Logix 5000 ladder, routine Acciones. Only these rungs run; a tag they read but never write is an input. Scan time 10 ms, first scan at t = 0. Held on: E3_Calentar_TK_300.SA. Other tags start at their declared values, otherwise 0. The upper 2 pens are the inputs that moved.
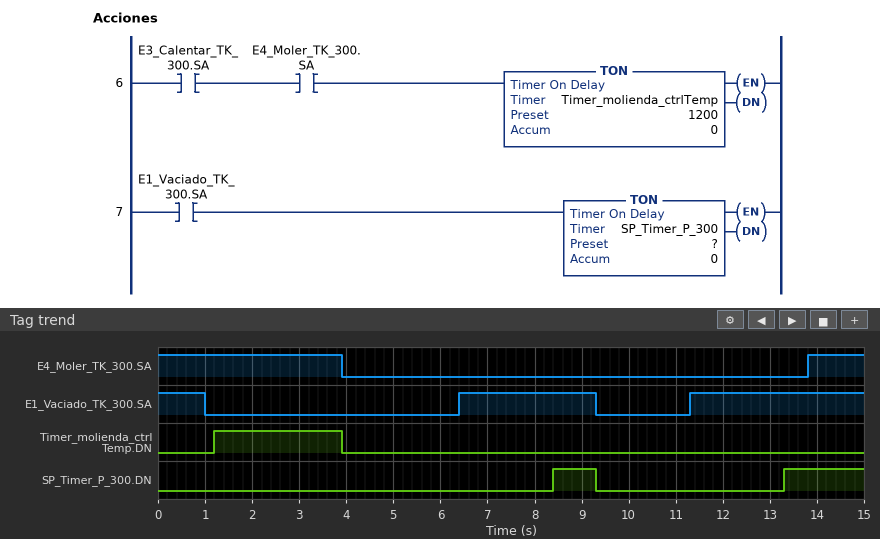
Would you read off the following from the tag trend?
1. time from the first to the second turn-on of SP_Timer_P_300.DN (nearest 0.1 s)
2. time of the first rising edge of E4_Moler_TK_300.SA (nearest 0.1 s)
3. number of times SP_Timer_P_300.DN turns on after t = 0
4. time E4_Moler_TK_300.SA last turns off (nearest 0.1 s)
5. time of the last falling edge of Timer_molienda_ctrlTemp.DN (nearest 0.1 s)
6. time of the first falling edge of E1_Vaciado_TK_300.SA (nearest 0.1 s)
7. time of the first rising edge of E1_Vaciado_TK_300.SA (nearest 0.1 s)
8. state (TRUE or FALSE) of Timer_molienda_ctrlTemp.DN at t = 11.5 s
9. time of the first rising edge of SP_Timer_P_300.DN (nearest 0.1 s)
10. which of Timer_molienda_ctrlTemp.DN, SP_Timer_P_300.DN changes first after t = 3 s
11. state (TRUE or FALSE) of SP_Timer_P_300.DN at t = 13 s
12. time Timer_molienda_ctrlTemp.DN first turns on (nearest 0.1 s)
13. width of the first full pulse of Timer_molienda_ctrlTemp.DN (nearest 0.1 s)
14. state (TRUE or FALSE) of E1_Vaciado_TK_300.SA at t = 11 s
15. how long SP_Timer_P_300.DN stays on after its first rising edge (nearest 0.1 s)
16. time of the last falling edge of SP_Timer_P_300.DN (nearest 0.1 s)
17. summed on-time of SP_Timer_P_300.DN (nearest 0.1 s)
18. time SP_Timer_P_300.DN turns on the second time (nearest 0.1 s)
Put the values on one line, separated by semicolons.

4.9 s; 13.8 s; 2; 3.9 s; 3.9 s; 1.0 s; 6.4 s; FALSE; 8.4 s; Timer_molienda_ctrlTemp.DN; FALSE; 1.2 s; 2.7 s; FALSE; 0.9 s; 9.3 s; 2.6 s; 13.3 s
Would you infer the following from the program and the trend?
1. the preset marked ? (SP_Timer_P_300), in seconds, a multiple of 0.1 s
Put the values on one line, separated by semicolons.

2.0 s
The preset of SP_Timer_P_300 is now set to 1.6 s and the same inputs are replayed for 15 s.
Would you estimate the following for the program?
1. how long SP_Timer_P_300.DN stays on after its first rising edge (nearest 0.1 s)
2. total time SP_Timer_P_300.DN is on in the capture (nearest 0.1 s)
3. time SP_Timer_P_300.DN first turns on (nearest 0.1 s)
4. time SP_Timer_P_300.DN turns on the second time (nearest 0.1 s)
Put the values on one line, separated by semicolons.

1.3 s; 3.4 s; 8.0 s; 12.9 s
